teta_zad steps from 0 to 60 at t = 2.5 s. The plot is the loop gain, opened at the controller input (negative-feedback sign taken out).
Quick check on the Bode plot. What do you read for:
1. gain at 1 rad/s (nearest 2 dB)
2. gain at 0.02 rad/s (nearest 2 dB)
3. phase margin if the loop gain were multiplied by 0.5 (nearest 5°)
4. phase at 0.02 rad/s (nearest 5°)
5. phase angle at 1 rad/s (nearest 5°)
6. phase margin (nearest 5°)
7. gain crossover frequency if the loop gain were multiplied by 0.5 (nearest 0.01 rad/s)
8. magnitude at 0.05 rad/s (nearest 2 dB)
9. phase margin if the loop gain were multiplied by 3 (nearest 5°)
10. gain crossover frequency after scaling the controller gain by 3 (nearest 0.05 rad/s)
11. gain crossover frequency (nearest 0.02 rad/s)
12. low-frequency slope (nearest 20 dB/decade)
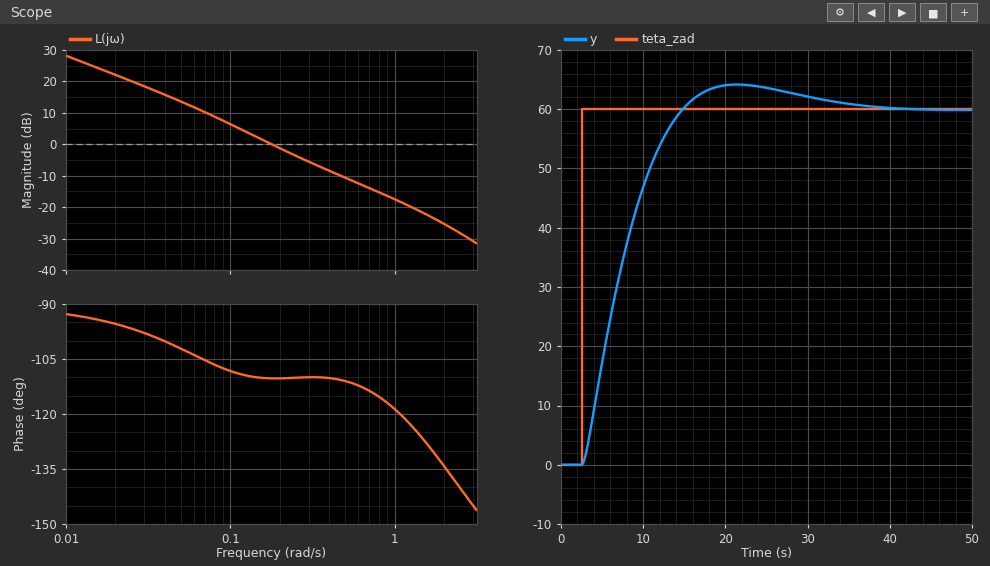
-18 dB
22 dB
70°
-95°
-120°
70°
0.10 rad/s
14 dB
70°
0.45 rad/s
0.18 rad/s
-20 dB/decade
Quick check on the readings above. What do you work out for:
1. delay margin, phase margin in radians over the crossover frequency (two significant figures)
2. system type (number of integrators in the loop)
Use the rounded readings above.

6.8 s
1
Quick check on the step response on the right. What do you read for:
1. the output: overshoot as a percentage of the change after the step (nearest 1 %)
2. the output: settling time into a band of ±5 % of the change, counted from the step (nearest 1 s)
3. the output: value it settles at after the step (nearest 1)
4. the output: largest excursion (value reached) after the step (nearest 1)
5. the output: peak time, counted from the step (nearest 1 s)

7 %
25 s
60
64
19 s
